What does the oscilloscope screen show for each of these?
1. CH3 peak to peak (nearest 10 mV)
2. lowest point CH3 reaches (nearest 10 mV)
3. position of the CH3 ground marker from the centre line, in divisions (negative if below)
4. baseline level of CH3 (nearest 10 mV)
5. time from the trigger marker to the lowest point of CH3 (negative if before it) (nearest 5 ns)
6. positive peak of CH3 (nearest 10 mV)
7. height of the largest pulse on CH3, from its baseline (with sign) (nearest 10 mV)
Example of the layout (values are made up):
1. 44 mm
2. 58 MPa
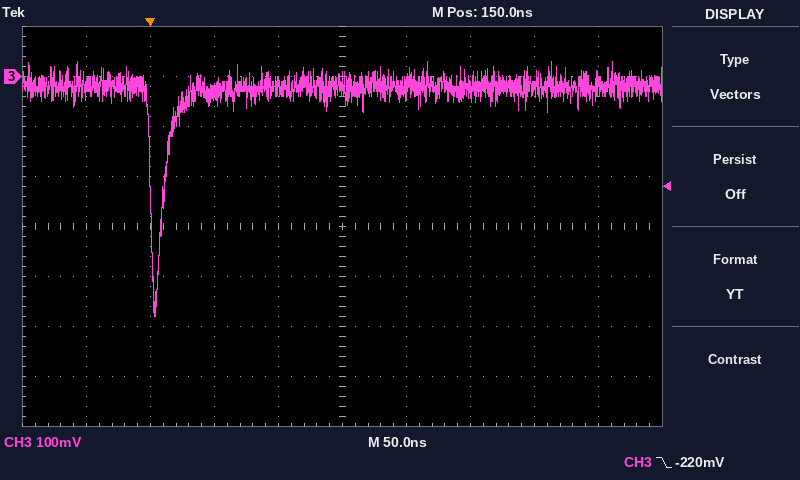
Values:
1. 510 mV
2. -480 mV
3. +3.0 div
4. -20 mV
5. +5 ns
6. 30 mV
7. -460 mV
